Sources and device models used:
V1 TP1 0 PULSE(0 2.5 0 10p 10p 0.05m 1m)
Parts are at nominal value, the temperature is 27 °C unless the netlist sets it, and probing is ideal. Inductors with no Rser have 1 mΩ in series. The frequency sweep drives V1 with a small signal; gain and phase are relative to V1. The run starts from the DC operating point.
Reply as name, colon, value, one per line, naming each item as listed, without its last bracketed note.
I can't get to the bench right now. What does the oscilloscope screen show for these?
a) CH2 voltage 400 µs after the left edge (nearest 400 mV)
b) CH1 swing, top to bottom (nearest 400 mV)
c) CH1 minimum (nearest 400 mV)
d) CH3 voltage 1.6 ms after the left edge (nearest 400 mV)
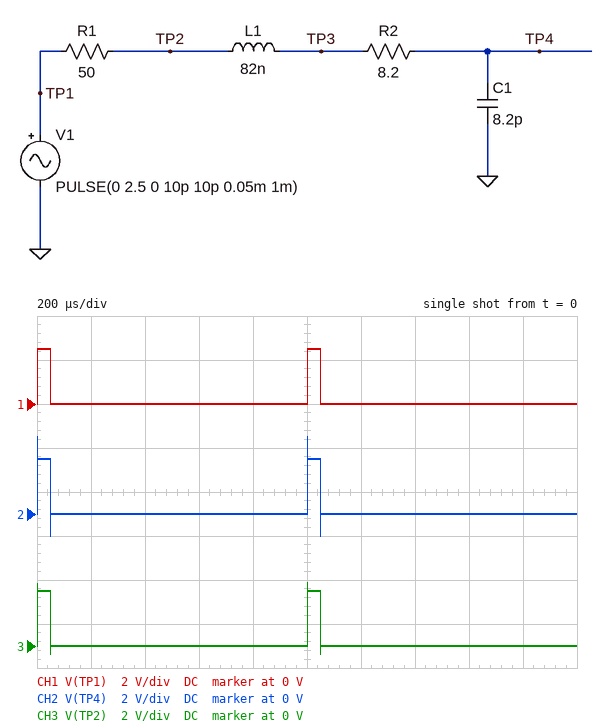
CH2 voltage 400 µs after the left edge: 0 V
CH1 swing, top to bottom: 2.4 V
CH1 minimum: 0 V
CH3 voltage 1.6 ms after the left edge: 0 V
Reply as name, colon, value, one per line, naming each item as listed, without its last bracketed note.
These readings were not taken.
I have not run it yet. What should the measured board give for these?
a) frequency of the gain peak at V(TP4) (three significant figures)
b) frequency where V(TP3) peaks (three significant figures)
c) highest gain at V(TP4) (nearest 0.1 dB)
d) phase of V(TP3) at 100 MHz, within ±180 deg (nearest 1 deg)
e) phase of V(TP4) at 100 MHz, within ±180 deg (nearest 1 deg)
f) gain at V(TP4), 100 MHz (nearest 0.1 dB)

frequency of the gain peak at V(TP4): 177 MHz
frequency where V(TP3) peaks: 177 MHz
highest gain at V(TP4): 5.1 dB
phase of V(TP3) at 100 MHz, within ±180 deg: -20 deg
phase of V(TP4) at 100 MHz, within ±180 deg: -22 deg
gain at V(TP4), 100 MHz: 2.0 dB
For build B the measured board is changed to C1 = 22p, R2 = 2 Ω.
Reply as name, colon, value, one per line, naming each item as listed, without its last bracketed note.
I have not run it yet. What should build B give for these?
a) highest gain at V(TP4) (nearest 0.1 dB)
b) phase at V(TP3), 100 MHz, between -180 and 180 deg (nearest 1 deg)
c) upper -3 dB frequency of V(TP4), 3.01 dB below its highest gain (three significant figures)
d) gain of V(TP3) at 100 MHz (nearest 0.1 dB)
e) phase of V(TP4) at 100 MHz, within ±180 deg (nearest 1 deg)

highest gain at V(TP4): 2.3 dB
phase at V(TP3), 100 MHz, between -180 and 180 deg: -67 deg
upper -3 dB frequency of V(TP4), 3.01 dB below its highest gain: 141 MHz
gain of V(TP3) at 100 MHz: 2.2 dB
phase of V(TP4) at 100 MHz, within ±180 deg: -68 deg
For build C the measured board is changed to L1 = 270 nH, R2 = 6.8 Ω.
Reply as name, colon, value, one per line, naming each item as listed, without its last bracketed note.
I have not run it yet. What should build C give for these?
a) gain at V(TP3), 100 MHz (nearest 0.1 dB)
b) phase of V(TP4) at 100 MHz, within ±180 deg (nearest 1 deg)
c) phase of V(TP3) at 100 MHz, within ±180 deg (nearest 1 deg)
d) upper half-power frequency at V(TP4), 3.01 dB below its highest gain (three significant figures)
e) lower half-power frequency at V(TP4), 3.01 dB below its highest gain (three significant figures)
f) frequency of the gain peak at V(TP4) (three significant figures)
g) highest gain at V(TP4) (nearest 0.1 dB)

gain at V(TP3), 100 MHz: 9.9 dB
phase of V(TP4) at 100 MHz, within ±180 deg: -67 deg
phase of V(TP3) at 100 MHz, within ±180 deg: -65 deg
upper half-power frequency at V(TP4), 3.01 dB below its highest gain: 120 MHz
lower half-power frequency at V(TP4), 3.01 dB below its highest gain: 85.7 MHz
frequency of the gain peak at V(TP4): 104 MHz
highest gain at V(TP4): 10.2 dB
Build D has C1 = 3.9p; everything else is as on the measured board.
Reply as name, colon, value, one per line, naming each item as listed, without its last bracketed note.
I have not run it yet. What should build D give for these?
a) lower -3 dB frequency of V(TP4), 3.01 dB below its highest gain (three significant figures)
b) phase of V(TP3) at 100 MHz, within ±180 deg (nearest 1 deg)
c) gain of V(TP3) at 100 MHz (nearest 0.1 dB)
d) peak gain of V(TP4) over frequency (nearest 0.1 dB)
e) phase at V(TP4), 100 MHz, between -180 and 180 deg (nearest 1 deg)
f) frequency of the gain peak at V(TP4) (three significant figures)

lower -3 dB frequency of V(TP4), 3.01 dB below its highest gain: 204 MHz
phase of V(TP3) at 100 MHz, within ±180 deg: -8 deg
gain of V(TP3) at 100 MHz: 1.1 dB
peak gain of V(TP4) over frequency: 8.1 dB
phase at V(TP4), 100 MHz, between -180 and 180 deg: -9 deg
frequency of the gain peak at V(TP4): 270 MHz
